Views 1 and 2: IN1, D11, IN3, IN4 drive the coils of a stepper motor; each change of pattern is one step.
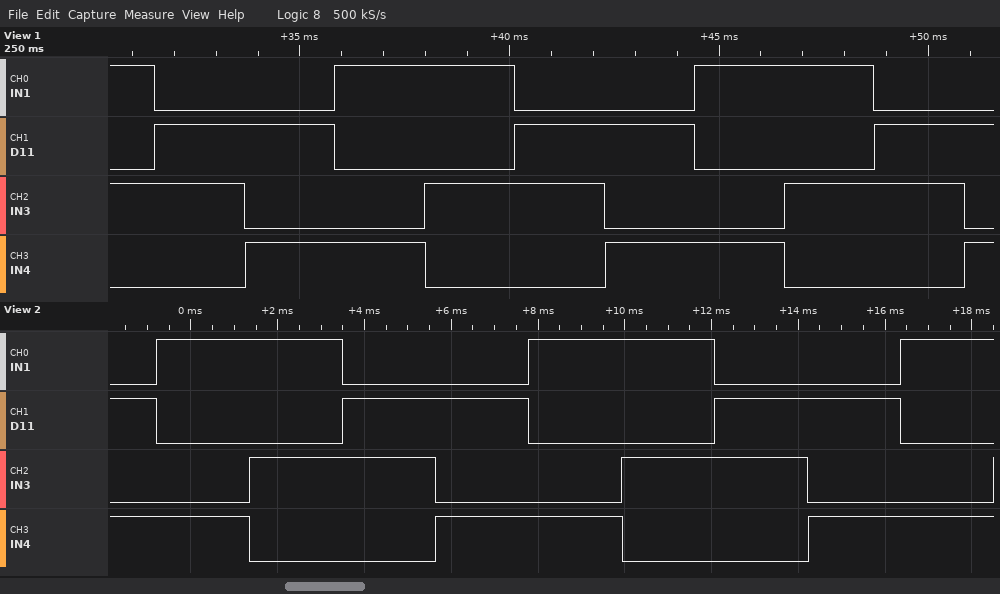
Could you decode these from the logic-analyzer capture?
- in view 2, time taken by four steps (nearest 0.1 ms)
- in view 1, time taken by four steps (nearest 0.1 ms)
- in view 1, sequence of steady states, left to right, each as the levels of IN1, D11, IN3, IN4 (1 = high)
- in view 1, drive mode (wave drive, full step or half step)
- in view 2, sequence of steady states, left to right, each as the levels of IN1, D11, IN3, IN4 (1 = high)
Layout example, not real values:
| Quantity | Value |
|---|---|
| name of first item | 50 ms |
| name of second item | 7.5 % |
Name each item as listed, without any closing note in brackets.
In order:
| Quantity | Value |
|---|---|
| in view 2, time taken by four steps | 8.6 ms |
| in view 1, time taken by four steps | 8.6 ms |
| in view 1, sequence of steady states, left to right, each as the levels of IN1, D11, IN3, IN4 | 1010 0110 0101 1001 1010 0110 0101 1001 1010 0110 0101 |
| in view 1, drive mode | full step |
| in view 2, sequence of steady states, left to right, each as the levels of IN1, D11, IN3, IN4 | 0101 1001 1010 0110 0101 1001 1010 0110 0101 1001 |
